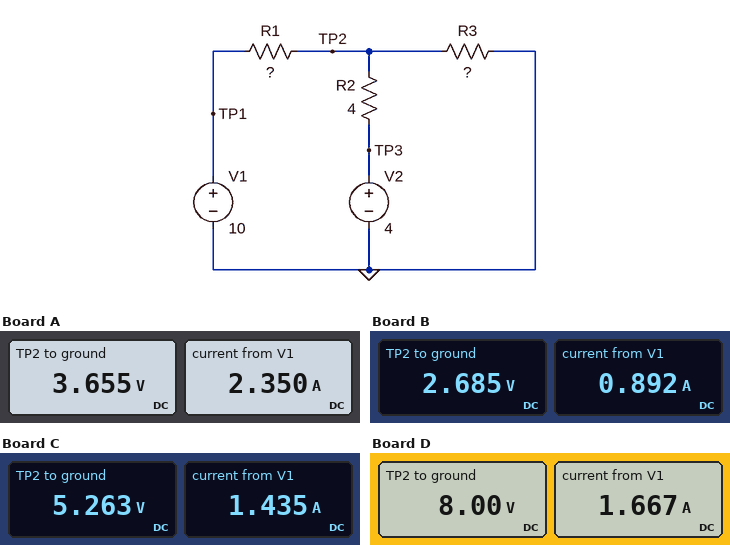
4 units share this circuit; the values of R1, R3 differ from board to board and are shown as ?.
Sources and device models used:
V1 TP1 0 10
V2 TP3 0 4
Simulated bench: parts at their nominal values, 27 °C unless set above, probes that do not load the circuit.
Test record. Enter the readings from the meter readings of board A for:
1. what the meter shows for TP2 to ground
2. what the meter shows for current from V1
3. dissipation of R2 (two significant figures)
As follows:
3.655 V
2.350 A
30 mW
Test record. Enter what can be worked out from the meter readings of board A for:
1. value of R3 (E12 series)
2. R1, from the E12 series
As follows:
1.5 Ω
2.7 Ω
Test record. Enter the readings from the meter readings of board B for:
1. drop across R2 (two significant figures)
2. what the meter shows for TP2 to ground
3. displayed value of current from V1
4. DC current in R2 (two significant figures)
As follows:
1.3 V
2.685 V
0.892 A
330 mA
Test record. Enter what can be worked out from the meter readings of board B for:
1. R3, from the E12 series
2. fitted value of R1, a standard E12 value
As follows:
2.2 Ω
8.2 Ω
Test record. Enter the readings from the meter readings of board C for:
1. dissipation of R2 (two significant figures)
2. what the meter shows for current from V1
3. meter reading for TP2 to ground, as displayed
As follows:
400 mW
1.435 A
5.263 V
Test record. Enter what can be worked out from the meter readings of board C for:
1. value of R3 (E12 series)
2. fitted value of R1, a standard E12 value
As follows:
4.7 Ω
3.3 Ω
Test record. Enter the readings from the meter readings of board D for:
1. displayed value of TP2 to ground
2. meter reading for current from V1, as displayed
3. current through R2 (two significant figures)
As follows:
8.00 V
1.667 A
1.0 A
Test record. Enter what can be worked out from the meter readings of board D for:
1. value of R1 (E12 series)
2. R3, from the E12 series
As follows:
1.2 Ω
12 Ω
